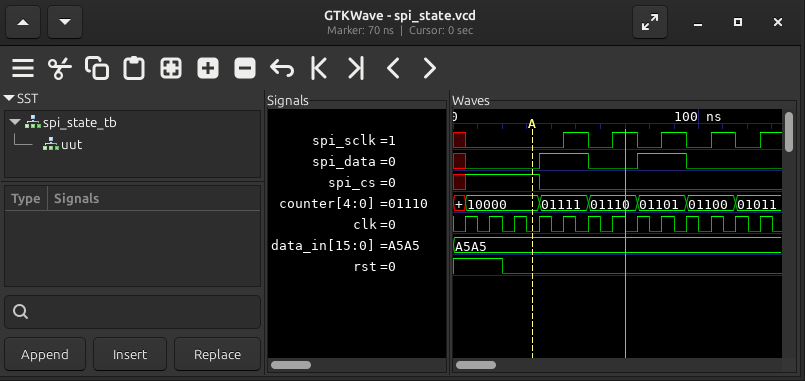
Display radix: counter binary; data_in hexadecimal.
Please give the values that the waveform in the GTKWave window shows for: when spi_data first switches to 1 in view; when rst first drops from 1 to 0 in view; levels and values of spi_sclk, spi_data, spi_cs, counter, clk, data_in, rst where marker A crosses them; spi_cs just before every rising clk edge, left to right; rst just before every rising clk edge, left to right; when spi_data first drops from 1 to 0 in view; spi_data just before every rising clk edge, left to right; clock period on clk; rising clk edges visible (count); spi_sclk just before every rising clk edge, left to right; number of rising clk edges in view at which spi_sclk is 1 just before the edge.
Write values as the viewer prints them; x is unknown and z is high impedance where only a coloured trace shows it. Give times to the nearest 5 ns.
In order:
35 ns
20 ns
spi_sclk=0, spi_data=0, spi_cs=1, counter=10000, clk=0, data_in=A5A5, rst=0
x 1 1 1 0 0 0 0 0 0 0 0 0
1 1 0 0 0 0 0 0 0 0 0 0 0
55 ns
x 0 0 0 1 1 0 0 1 1 0 0 0
10 ns
13
x 0 0 0 0 1 0 1 0 1 0 1 0
4
